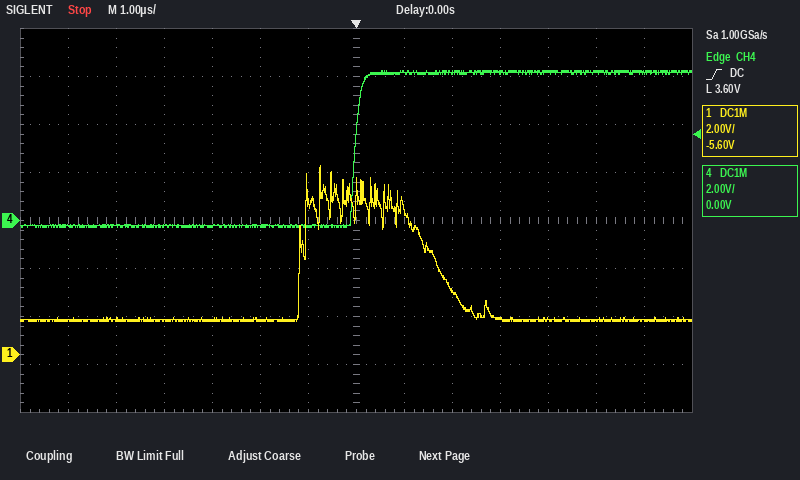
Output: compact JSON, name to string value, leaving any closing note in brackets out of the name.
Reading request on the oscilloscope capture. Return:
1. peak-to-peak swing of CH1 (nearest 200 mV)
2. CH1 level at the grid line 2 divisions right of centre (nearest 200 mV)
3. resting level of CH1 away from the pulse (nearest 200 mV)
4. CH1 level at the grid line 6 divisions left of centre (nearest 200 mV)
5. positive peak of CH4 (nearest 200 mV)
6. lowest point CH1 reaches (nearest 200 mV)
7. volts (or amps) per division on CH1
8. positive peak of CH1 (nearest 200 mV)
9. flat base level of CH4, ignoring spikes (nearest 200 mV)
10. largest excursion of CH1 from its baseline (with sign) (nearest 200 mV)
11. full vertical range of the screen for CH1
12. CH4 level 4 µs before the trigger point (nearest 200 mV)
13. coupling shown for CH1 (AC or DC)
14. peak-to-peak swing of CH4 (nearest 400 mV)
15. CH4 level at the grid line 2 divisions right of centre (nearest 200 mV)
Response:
{"peak-to-peak swing of CH1": "6.4 V", "CH1 level at the grid line 2 divisions right of centre": "2.6 V", "resting level of CH1 away from the pulse": "1.4 V", "CH1 level at the grid line 6 divisions left of centre": "1.4 V", "positive peak of CH4": "6.2 V", "lowest point CH1 reaches": "1.4 V", "volts (or amps) per division on CH1": "2 V", "positive peak of CH1": "7.8 V", "flat base level of CH4, ignoring spikes": "-200 mV", "largest excursion of CH1 from its baseline (with sign)": "+6.4 V", "full vertical range of the screen for CH1": "16 V", "CH4 level 4 µs before the trigger point": "-200 mV", "coupling shown for CH1": "DC", "peak-to-peak swing of CH4": "6.4 V", "CH4 level at the grid line 2 divisions right of centre": "6.2 V"}
